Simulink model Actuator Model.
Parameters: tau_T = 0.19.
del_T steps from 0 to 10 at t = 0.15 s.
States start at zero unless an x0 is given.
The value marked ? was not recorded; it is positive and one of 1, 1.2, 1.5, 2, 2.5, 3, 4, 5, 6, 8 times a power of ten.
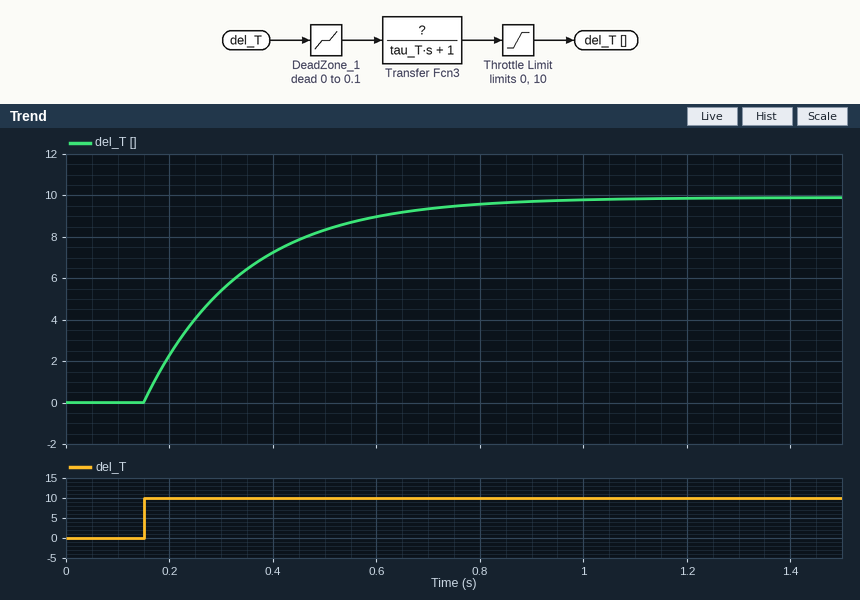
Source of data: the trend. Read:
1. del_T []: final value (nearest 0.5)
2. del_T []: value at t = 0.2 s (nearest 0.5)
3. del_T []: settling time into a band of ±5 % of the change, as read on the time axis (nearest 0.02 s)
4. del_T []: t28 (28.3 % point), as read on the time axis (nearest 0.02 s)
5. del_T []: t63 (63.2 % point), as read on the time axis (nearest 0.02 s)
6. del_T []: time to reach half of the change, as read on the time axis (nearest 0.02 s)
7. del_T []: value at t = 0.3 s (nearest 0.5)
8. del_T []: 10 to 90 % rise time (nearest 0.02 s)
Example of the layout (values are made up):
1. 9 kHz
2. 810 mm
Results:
1. 10.0
2. 2.5
3. 0.72 s
4. 0.22 s
5. 0.34 s
6. 0.28 s
7. 5.5
8. 0.42 s
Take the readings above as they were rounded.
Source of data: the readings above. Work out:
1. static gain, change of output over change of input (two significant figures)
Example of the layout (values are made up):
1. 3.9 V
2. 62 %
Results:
1. 1.0
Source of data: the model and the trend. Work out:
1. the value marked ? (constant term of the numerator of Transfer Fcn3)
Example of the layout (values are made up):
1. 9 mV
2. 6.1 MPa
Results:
1. 1
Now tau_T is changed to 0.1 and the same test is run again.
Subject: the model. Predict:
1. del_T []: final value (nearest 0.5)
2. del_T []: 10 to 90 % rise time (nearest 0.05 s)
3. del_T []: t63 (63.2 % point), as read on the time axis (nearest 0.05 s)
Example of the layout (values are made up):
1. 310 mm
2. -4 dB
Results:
1. 10.0
2. 0.20 s
3. 0.25 s
